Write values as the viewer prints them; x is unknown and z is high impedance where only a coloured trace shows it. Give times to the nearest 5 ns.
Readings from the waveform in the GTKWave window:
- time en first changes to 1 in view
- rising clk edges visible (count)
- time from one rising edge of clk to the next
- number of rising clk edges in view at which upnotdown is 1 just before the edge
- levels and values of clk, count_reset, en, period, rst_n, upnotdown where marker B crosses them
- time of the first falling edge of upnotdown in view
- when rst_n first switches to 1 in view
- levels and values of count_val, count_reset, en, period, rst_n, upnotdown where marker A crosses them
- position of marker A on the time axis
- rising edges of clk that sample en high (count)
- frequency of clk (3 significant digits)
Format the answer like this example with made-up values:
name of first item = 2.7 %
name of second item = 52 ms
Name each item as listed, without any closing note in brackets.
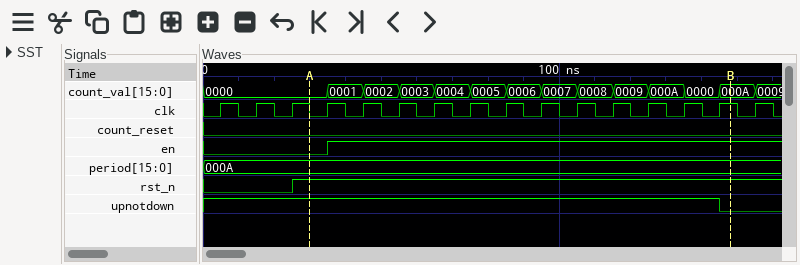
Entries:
time en first changes to 1 in view = 35 ns
rising clk edges visible = 16
time from one rising edge of clk to the next = 10 ns
number of rising clk edges in view at which upnotdown is 1 just before the edge = 15
levels and values of clk, count_reset, en, period, rst_n, upnotdown where marker B crosses them = clk=1, count_reset=0, en=1, period=000A, rst_n=1, upnotdown=0
time of the first falling edge of upnotdown in view = 145 ns
when rst_n first switches to 1 in view = 25 ns
levels and values of count_val, count_reset, en, period, rst_n, upnotdown where marker A crosses them = count_val=0000, count_reset=0, en=0, period=000A, rst_n=1, upnotdown=1
position of marker A on the time axis = 30 ns
rising edges of clk that sample en high = 12
frequency of clk = 100 MHz
